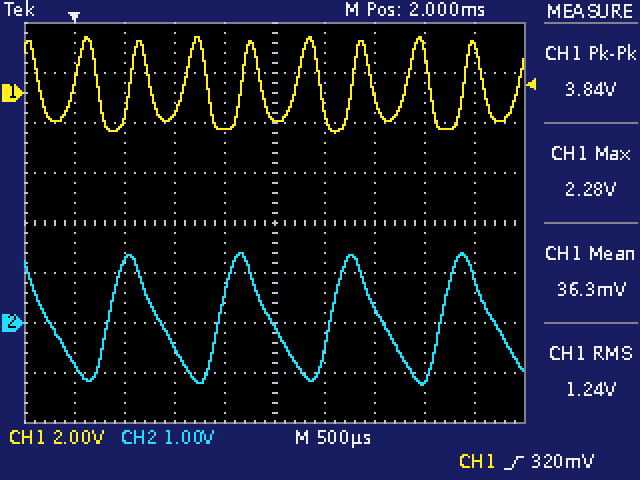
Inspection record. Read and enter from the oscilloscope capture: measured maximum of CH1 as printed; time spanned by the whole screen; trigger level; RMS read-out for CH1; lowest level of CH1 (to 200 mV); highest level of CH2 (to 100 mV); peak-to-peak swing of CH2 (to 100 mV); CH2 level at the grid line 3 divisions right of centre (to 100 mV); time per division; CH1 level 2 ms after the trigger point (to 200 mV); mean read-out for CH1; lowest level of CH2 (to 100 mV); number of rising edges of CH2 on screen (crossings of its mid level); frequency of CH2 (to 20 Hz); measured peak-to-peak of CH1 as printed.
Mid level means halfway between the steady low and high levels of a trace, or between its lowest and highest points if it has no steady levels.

2.28 V
5 ms
320 mV
1.24 V
-1.6 V
1.4 V
2.6 V
-1.1 V
500 µs
-1.0 V
36.3 mV
-1.2 V
4
900 Hz
3.84 V
